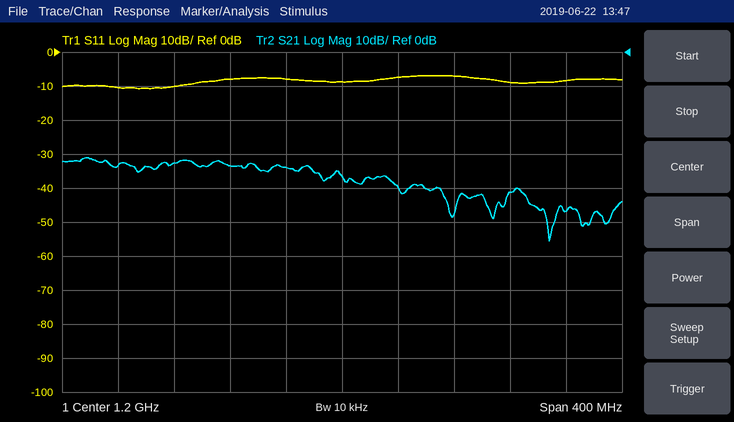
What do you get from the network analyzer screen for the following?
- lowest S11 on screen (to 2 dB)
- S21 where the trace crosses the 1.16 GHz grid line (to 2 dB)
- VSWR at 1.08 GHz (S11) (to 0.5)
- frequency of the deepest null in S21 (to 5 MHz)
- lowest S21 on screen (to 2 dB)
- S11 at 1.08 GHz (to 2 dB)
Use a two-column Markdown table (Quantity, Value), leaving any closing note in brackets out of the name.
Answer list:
| Quantity | Value |
|---|---|
| lowest S11 on screen | -10 dB |
| S21 where the trace crosses the 1.16 GHz grid line | -34 dB |
| VSWR at 1.08 GHz (S11) | 2.0 |
| frequency of the deepest null in S21 | 1.350 GHz |
| lowest S21 on screen | -56 dB |
| S11 at 1.08 GHz | -10 dB |
